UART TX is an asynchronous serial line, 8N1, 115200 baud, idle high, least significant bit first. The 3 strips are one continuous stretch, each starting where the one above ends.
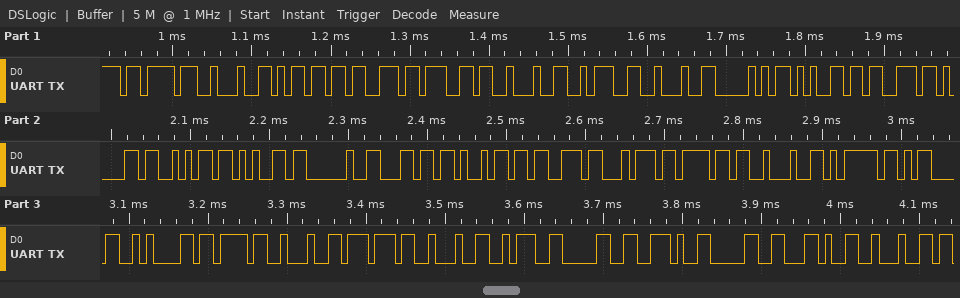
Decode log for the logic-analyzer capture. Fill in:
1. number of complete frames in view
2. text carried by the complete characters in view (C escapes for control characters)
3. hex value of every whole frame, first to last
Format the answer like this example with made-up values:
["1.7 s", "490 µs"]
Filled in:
["34", "\"{\\\"msg\\\":\\\"Pesaje listo\\\"}\\r\\n{\\\"w\\\":0.0,\\\"\"", "0x7B 0x22 0x6D 0x73 0x67 0x22 0x3A 0x22 0x50 0x65 0x73 0x61 0x6A 0x65 0x20 0x6C 0x69 0x73 0x74 0x6F 0x22 0x7D 0x0D 0x0A 0x7B 0x22 0x77 0x22 0x3A 0x30 0x2E 0x30 0x2C 0x22"]
